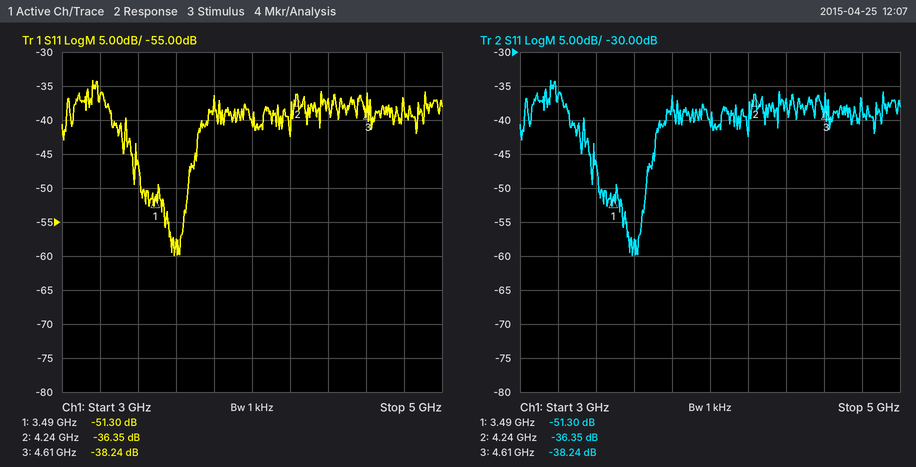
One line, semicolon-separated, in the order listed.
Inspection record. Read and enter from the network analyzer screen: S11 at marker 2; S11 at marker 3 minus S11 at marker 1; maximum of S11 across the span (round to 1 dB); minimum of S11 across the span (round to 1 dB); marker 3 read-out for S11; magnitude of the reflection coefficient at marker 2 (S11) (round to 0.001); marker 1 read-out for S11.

-36.35 dB; 13.06 dB; -34 dB; -60 dB; -38.24 dB; 0.015; -51.30 dB
